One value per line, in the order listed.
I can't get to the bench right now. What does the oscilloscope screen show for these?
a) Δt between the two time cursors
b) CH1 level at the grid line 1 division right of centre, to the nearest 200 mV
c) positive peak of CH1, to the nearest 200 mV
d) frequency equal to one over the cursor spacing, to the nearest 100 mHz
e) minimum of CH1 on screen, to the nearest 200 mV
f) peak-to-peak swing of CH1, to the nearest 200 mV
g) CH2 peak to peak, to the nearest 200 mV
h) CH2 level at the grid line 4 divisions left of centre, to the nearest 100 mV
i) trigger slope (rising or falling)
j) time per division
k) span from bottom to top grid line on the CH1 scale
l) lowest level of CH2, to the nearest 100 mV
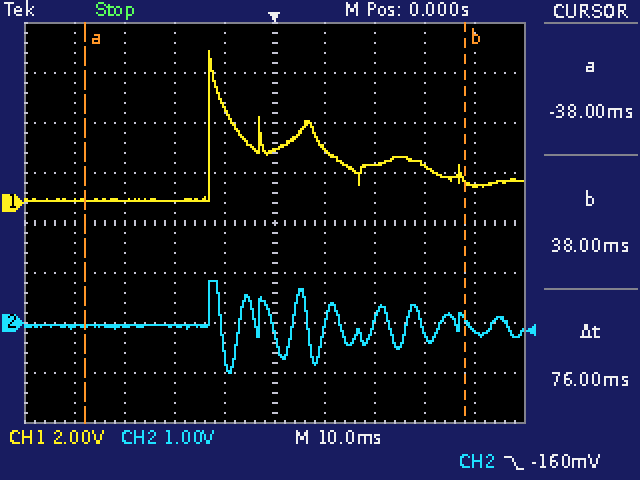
76 ms
2.2 V
6.0 V
13.2 Hz
0.0 V
6.0 V
1.8 V
-100 mV
falling
10 ms
16 V
-1.0 V
